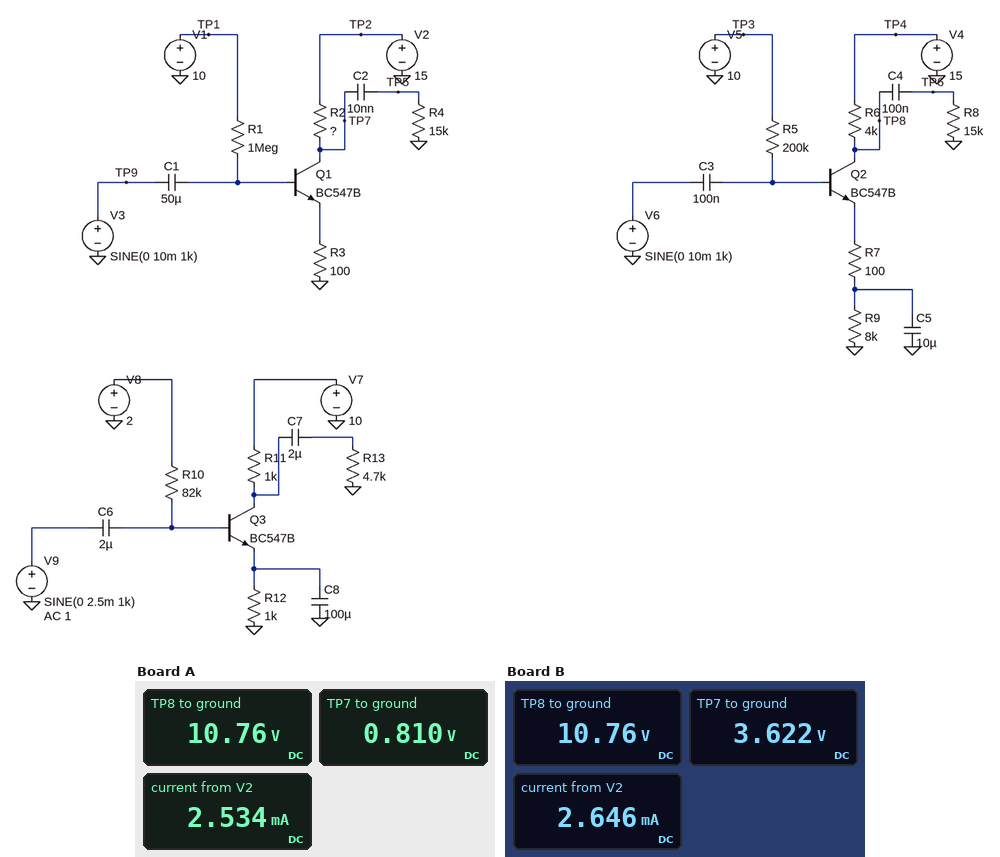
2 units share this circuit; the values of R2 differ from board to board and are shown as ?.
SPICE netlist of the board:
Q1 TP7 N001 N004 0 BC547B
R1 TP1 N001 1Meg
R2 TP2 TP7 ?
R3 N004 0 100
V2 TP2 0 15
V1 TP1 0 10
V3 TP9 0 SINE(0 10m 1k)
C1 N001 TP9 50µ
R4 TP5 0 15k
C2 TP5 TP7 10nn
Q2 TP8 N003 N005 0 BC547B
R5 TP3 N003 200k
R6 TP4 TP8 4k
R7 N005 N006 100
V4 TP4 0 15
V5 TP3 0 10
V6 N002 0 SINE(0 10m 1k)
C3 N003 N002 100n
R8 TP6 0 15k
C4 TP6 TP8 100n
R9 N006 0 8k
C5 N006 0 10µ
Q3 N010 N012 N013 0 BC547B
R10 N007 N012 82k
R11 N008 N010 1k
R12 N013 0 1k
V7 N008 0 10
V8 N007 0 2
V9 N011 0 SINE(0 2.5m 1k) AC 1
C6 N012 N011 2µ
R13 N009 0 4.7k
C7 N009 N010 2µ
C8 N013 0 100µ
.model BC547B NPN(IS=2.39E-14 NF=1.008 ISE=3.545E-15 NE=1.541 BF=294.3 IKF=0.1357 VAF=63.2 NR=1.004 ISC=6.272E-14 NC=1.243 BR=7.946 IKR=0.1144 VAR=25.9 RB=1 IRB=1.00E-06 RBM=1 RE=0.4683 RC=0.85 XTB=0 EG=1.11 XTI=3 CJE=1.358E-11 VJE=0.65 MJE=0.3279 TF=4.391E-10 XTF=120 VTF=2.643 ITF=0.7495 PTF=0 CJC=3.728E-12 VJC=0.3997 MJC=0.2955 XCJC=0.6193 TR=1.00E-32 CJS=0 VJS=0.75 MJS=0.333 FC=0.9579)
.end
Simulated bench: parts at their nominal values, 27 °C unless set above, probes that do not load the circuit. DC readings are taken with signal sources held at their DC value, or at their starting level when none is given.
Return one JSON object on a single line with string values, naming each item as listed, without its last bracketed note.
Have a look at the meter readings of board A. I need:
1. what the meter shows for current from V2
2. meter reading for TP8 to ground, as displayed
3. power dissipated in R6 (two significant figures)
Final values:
{"what the meter shows for current from V2": "2.534 mA", "meter reading for TP8 to ground, as displayed": "10.76 V", "power dissipated in R6": "4.5 mW"}
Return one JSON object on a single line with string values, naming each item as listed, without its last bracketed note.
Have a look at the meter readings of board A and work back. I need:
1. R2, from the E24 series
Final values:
{"R2, from the E24 series": "5.6 kΩ"}
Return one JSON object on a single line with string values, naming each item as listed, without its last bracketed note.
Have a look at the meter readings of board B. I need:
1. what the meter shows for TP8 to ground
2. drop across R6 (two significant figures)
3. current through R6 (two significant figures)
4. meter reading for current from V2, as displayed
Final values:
{"what the meter shows for TP8 to ground": "10.76 V", "drop across R6": "4.2 V", "current through R6": "1.1 mA", "meter reading for current from V2, as displayed": "2.646 mA"}
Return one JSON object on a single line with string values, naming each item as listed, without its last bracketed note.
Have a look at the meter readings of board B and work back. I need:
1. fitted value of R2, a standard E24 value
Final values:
{"fitted value of R2, a standard E24 value": "4.3 kΩ"}
